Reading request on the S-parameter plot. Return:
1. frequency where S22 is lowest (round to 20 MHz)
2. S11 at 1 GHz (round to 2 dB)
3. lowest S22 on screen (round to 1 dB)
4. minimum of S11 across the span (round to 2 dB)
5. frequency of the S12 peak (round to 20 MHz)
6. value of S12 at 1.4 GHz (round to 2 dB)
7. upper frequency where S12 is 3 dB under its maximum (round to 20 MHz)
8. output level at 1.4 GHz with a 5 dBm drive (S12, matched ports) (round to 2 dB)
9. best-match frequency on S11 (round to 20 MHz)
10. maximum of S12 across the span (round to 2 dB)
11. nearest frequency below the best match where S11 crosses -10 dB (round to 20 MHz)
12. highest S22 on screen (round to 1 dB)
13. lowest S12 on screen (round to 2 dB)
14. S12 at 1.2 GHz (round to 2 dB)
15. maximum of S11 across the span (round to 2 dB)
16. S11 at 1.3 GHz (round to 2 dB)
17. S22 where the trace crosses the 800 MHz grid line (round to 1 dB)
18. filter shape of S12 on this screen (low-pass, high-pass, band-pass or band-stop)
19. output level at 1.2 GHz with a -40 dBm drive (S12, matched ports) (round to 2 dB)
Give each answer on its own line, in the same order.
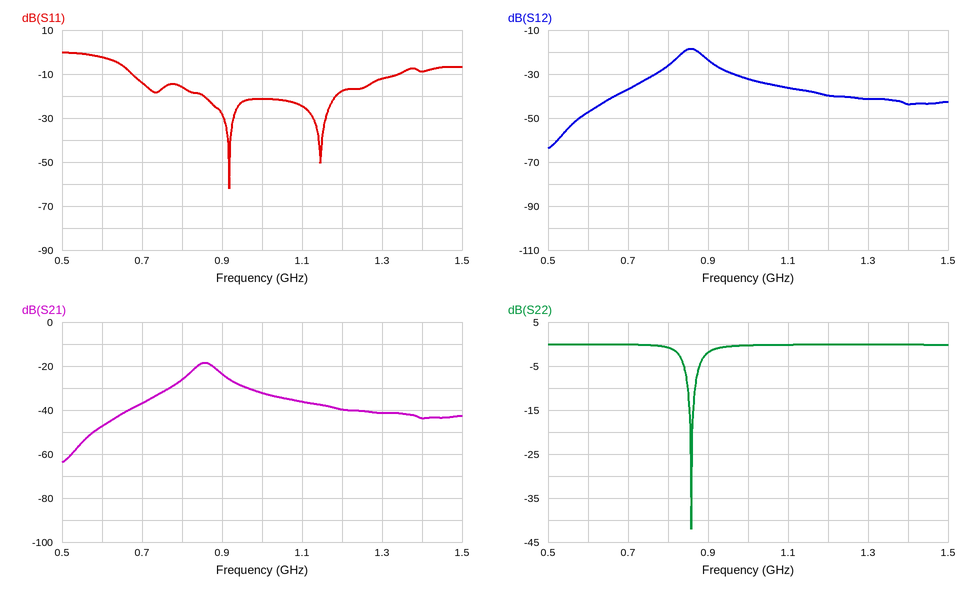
860 MHz
-22 dB
-42 dB
-62 dB
860 MHz
-44 dB
880 MHz
-38 dBm
920 MHz
-18 dB
680 MHz
0 dB
-64 dB
-40 dB
0 dB
-12 dB
-1 dB
band-pass
-80 dBm
